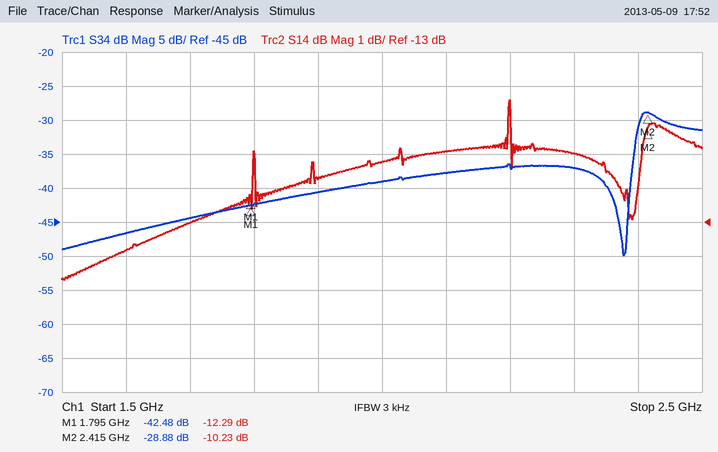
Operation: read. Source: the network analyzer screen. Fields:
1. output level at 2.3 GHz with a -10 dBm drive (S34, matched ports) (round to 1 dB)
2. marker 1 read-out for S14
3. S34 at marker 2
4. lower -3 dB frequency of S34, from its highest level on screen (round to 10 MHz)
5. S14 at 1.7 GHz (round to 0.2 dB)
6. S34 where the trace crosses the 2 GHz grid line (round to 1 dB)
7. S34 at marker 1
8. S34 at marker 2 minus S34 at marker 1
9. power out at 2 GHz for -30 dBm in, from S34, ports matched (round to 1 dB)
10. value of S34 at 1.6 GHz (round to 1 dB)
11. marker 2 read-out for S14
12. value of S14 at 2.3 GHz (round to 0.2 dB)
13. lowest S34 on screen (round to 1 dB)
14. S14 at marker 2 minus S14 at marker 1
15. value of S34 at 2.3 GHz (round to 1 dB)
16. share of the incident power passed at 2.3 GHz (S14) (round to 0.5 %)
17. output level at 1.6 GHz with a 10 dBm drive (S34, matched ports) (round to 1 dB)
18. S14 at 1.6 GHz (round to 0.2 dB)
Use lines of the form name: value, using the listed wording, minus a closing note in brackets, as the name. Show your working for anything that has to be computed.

output level at 2.3 GHz with a -10 dBm drive (S34, matched ports): -10 dBm + (-37 dB) = -47 dBm
marker 1 read-out for S14: -12.29 dB
S34 at marker 2: -28.88 dB
lower -3 dB frequency of S34, from its highest level on screen: 2.40 GHz
S14 at 1.7 GHz: -13.0 dB
S34 where the trace crosses the 2 GHz grid line: -39 dB
S34 at marker 1: -42.48 dB
S34 at marker 2 minus S34 at marker 1: -28.88 − (-42.48) = 13.60 dB
power out at 2 GHz for -30 dBm in, from S34, ports matched: -30 dBm + (-39 dB) = -69 dBm
value of S34 at 1.6 GHz: -47 dB
marker 2 read-out for S14: -10.23 dB
value of S14 at 2.3 GHz: -11.0 dB
lowest S34 on screen: -50 dB
S14 at marker 2 minus S14 at marker 1: -10.23 − (-12.29) = 2.06 dB
value of S34 at 2.3 GHz: -37 dB
share of the incident power passed at 2.3 GHz (S14): 10^(-11/10) ≈ 7.94 %, so 8.0 % to the nearest 0.5 %
output level at 1.6 GHz with a 10 dBm drive (S34, matched ports): 10 dBm + (-47 dB) = -37 dBm
S14 at 1.6 GHz: -13.8 dB
